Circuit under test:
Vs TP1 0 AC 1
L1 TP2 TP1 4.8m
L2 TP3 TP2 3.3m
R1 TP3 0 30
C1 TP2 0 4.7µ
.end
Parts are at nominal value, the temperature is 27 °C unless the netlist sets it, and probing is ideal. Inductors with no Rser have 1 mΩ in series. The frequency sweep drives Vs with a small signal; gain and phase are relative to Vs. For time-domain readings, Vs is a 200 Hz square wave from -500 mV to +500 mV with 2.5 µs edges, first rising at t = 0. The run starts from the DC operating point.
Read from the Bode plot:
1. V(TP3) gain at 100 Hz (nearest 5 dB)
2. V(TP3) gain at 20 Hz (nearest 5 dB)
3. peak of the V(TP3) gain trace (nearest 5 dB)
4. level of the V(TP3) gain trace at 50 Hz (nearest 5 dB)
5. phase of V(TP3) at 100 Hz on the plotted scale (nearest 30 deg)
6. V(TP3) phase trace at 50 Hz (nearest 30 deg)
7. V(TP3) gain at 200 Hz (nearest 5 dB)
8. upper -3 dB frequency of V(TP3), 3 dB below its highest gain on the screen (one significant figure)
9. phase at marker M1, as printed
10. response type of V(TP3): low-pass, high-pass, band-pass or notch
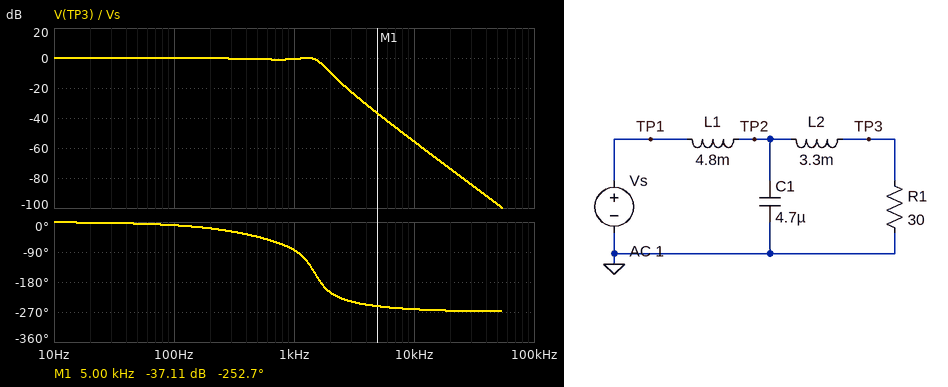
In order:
0 dB
0 dB
0 dB
0 dB
0 deg
0 deg
0 dB
2 kHz
-252.7 deg
low-pass
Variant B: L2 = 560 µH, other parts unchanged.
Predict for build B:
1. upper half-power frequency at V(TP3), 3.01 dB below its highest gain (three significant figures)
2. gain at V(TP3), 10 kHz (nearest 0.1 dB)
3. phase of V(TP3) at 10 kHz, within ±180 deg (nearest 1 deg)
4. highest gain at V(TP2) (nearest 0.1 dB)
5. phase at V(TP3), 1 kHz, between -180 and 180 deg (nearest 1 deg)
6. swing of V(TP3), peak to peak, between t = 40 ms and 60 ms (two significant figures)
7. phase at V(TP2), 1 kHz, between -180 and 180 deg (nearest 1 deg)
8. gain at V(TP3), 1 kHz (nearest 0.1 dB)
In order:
1.30 kHz
-42.2 dB
133 deg
0.6 dB
-84 deg
1.2 V
-77 deg
-0.2 dB
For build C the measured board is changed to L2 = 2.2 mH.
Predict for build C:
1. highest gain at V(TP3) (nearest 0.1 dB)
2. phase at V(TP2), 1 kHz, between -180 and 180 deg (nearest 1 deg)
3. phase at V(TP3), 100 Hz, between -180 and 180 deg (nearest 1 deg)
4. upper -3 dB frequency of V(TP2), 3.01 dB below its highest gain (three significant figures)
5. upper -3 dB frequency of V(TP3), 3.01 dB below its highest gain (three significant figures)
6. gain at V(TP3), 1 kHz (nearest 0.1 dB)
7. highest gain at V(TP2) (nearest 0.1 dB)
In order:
0 dB
-59 deg
-8 deg
1.73 kHz
1.58 kHz
-0.5 dB
0.4 dB
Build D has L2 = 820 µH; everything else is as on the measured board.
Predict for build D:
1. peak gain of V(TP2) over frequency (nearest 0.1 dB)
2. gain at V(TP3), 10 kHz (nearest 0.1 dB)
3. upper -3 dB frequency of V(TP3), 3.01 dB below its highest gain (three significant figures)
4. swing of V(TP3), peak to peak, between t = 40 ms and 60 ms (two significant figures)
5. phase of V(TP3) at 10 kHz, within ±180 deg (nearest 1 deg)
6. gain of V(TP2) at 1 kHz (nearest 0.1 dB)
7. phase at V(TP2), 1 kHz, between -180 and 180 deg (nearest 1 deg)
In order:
0.5 dB
-44.4 dB
1.34 kHz
1.2 V
122 deg
-0.1 dB
-74 deg
